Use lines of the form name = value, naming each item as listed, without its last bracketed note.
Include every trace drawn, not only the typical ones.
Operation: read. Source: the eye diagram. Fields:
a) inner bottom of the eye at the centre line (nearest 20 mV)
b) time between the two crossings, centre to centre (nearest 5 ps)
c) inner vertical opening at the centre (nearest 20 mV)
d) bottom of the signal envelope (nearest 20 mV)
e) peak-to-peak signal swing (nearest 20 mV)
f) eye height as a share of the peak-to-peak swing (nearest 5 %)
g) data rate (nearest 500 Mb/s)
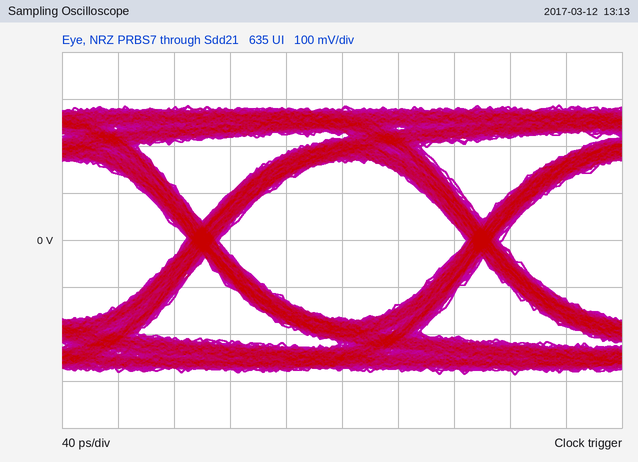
inner bottom of the eye at the centre line = -160 mV
time between the two crossings, centre to centre = 200 ps
inner vertical opening at the centre = 340 mV
bottom of the signal envelope = -280 mV
peak-to-peak signal swing = 580 mV
eye height as a share of the peak-to-peak swing = 60 %
data rate = 5.0 Gb/s
